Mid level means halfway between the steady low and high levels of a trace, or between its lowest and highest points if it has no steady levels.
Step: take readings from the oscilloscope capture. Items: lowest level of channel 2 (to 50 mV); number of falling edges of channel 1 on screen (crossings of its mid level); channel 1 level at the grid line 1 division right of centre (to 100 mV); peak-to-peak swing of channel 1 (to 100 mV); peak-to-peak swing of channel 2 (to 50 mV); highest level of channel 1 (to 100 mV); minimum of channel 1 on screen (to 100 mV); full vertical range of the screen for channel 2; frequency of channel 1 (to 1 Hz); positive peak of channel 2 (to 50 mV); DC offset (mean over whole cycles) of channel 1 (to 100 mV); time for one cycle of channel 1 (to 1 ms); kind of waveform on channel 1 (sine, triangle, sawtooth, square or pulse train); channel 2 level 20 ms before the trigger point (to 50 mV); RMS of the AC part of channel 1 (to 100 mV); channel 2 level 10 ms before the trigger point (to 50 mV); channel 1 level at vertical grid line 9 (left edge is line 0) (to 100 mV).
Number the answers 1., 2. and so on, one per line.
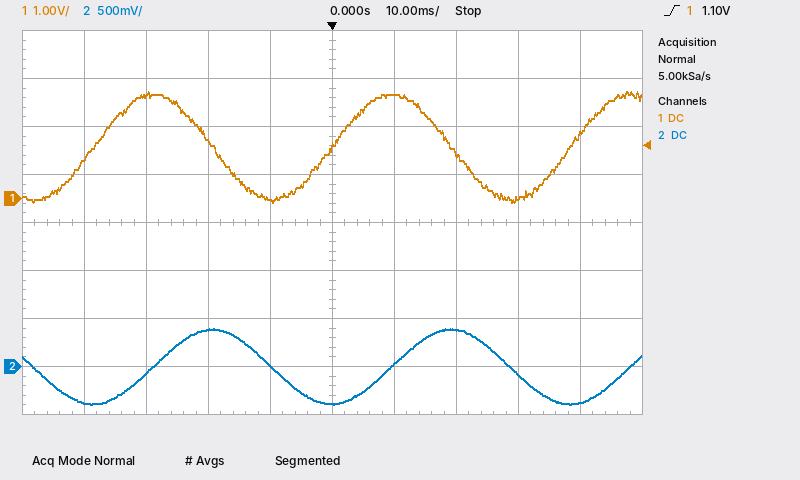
1. -400 mV
2. 2
3. 2.2 V
4. 2.3 V
5. 800 mV
6. 2.2 V
7. -100 mV
8. 4 V
9. 26 Hz
10. 400 mV
11. 1.1 V
12. 38 ms
13. sine
14. 400 mV
15. 800 mV
16. 0 mV
17. 1.3 V
